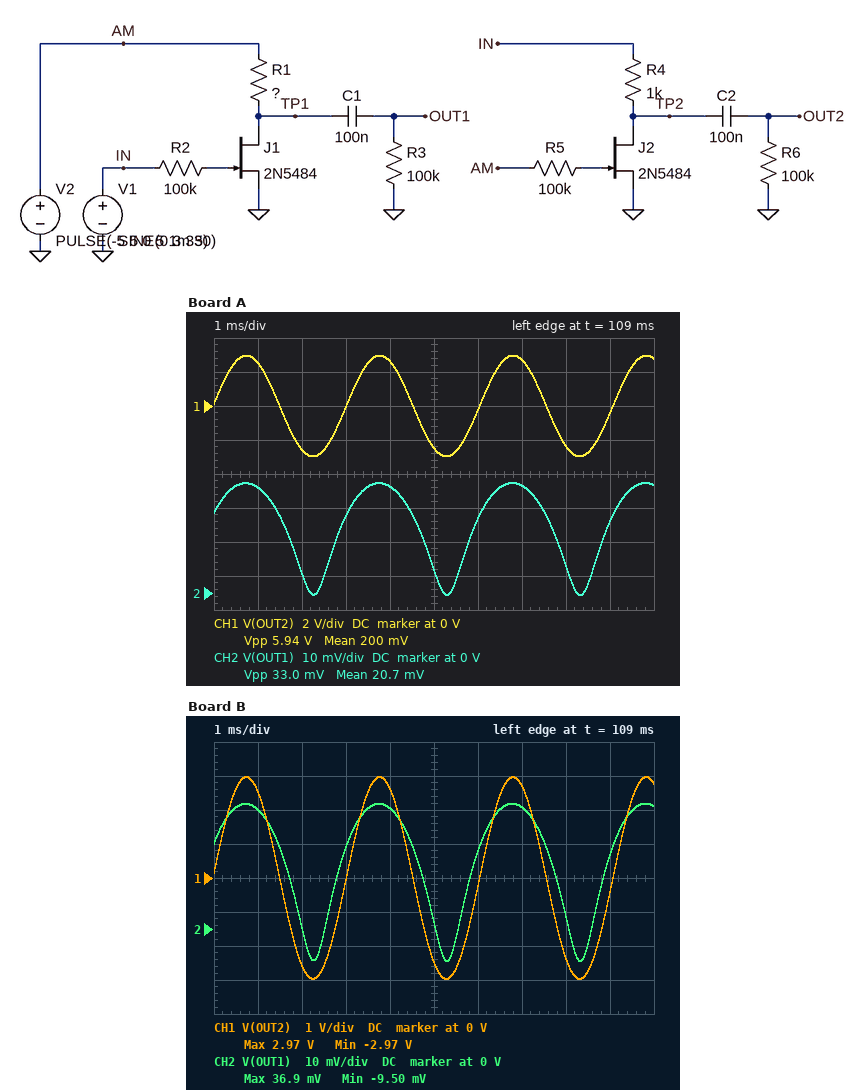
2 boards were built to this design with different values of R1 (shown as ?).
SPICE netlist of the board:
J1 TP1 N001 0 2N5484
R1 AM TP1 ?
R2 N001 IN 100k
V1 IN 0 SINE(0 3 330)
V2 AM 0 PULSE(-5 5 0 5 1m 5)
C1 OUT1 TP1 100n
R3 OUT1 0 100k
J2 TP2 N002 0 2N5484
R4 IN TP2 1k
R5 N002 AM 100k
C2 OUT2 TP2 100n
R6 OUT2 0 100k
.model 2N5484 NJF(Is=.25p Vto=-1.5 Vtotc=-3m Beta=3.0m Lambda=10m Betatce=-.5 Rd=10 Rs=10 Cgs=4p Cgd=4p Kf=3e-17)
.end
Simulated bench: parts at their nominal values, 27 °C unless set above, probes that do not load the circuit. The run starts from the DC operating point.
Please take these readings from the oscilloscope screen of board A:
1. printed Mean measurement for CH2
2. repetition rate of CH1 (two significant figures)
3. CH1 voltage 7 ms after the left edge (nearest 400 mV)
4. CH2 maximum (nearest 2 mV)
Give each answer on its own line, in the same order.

20.7 mV
330 Hz
2.8 V
32 mV
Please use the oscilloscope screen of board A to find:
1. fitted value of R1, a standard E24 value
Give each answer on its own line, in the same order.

43 Ω
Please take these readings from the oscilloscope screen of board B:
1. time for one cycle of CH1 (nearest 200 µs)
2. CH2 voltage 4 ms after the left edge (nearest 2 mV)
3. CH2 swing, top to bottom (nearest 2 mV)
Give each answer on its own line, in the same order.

3.0 ms
36 mV
46 mV
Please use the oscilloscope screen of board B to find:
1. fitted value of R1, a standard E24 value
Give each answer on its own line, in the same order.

56 Ω
